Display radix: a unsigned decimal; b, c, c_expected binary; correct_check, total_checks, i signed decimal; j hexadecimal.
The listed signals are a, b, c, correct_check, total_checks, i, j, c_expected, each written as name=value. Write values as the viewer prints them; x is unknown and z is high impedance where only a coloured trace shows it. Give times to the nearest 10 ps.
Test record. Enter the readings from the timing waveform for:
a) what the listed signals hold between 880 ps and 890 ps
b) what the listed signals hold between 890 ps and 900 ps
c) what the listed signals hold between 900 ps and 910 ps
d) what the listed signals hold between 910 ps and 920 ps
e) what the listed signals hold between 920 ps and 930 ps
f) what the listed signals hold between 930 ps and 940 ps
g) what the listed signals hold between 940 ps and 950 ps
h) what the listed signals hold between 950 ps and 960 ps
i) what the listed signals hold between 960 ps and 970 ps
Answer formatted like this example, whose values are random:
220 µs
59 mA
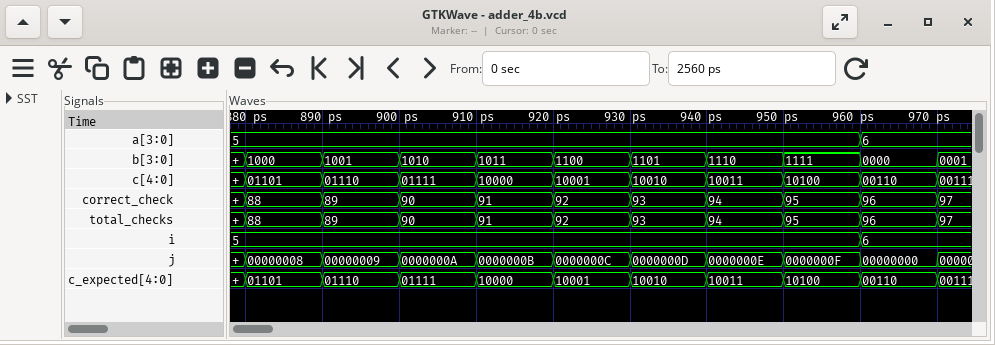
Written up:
a=5, b=1000, c=01101, correct_check=88, total_checks=88, i=5, j=00000008, c_expected=01101
a=5, b=1001, c=01110, correct_check=89, total_checks=89, i=5, j=00000009, c_expected=01110
a=5, b=1010, c=01111, correct_check=90, total_checks=90, i=5, j=0000000A, c_expected=01111
a=5, b=1011, c=10000, correct_check=91, total_checks=91, i=5, j=0000000B, c_expected=10000
a=5, b=1100, c=10001, correct_check=92, total_checks=92, i=5, j=0000000C, c_expected=10001
a=5, b=1101, c=10010, correct_check=93, total_checks=93, i=5, j=0000000D, c_expected=10010
a=5, b=1110, c=10011, correct_check=94, total_checks=94, i=5, j=0000000E, c_expected=10011
a=5, b=1111, c=10100, correct_check=95, total_checks=95, i=5, j=0000000F, c_expected=10100
a=6, b=0000, c=00110, correct_check=96, total_checks=96, i=6, j=00000000, c_expected=00110
